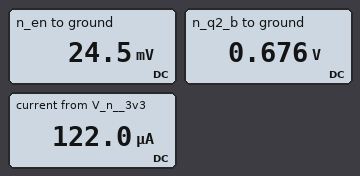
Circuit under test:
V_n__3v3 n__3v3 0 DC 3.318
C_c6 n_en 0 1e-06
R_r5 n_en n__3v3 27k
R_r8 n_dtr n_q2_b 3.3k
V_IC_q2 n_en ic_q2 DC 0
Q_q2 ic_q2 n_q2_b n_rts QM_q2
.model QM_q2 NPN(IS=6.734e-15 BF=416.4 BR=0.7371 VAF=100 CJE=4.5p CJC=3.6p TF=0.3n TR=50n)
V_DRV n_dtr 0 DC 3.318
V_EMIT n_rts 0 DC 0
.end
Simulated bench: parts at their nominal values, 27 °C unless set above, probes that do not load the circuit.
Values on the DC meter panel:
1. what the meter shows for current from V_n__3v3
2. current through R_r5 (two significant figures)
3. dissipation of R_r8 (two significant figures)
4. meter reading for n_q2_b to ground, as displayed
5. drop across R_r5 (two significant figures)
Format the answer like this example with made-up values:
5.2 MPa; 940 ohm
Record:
122.0 µA; 120 µA; 2.1 mW; 0.676 V; 3.3 V
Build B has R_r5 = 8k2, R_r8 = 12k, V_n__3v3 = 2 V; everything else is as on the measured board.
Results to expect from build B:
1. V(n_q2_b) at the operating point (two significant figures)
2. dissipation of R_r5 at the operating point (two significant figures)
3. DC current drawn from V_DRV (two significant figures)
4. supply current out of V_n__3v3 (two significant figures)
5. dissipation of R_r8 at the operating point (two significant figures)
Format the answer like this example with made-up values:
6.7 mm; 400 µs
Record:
650 mV; 470 µW; 220 µA; 240 µA; 590 µW
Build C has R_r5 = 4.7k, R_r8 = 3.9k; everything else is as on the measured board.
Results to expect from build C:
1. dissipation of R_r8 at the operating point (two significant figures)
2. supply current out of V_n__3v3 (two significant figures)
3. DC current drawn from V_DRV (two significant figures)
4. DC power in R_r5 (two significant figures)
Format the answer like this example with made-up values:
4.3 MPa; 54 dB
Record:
1.8 mW; 700 µA; 680 µA; 2.3 mW
